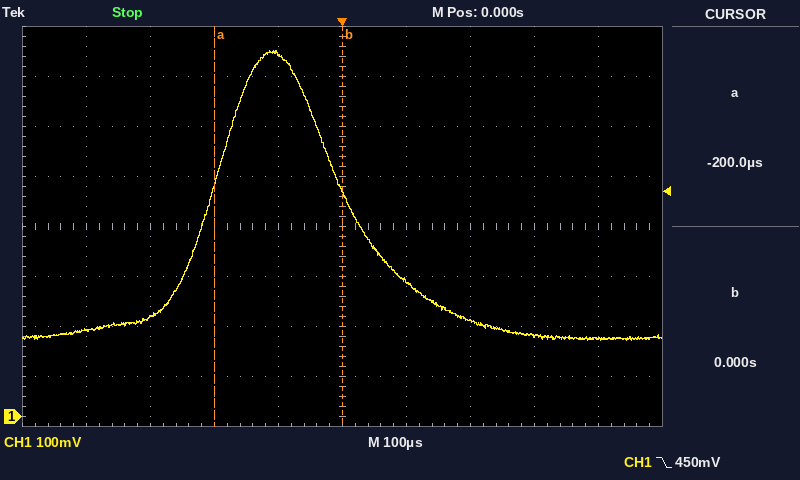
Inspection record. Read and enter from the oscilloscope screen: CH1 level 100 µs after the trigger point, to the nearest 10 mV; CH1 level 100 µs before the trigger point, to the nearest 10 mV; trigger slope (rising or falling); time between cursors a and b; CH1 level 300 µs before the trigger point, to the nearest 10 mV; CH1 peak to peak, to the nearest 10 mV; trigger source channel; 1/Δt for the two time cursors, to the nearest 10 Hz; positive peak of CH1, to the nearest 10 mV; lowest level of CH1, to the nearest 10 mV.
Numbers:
270 mV
730 mV
falling
200 µs
200 mV
580 mV
CH1
5.00 kHz
730 mV
150 mV
